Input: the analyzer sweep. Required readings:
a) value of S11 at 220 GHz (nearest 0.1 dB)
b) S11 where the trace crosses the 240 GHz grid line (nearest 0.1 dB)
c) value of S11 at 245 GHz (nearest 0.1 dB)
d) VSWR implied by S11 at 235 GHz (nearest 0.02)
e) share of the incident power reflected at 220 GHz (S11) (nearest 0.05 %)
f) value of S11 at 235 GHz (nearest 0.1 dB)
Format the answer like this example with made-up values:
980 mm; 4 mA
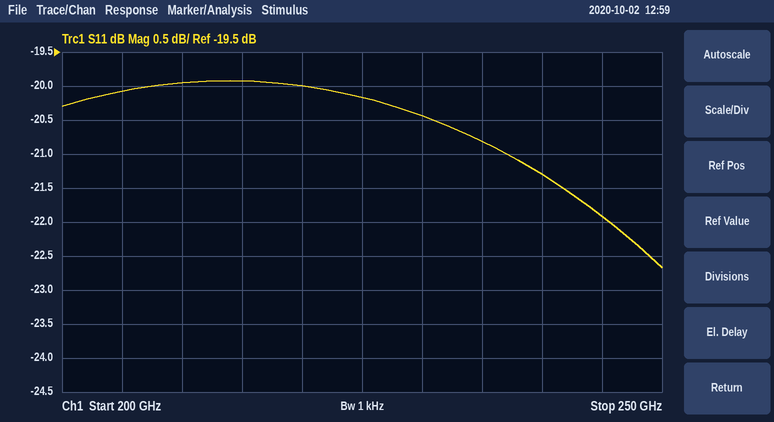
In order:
-20.0 dB; -21.3 dB; -21.9 dB; 1.20; 1.00 %; -20.8 dB
